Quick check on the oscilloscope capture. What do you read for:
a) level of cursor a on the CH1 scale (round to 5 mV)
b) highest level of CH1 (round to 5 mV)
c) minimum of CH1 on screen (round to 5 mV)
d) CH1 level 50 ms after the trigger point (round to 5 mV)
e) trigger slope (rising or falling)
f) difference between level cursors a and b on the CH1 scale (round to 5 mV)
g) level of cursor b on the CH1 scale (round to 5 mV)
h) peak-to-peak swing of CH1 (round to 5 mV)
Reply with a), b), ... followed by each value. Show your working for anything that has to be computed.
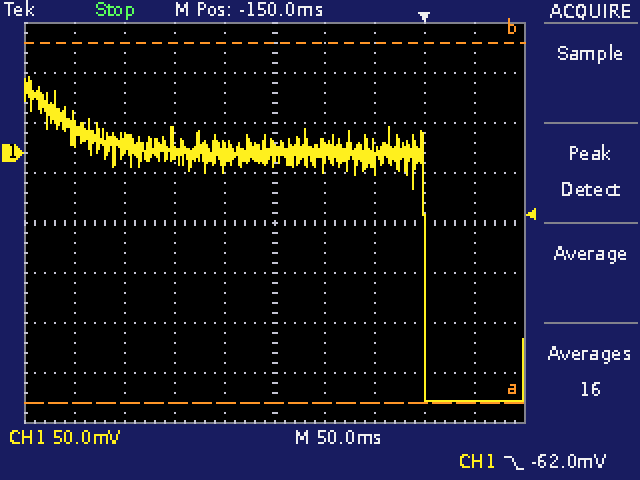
a) -250 mV
b) 75 mV
c) -250 mV
d) -250 mV
e) falling
f) 360 mV
g) 110 mV
h) 75 mV − (-250 mV) = 325 mV
